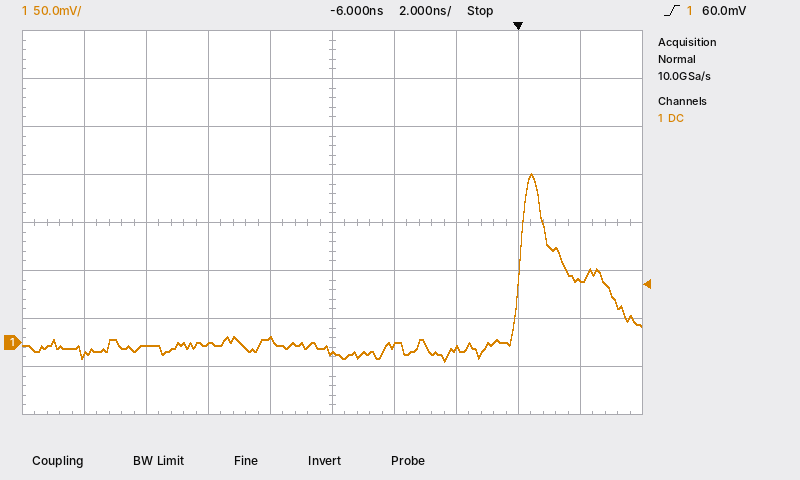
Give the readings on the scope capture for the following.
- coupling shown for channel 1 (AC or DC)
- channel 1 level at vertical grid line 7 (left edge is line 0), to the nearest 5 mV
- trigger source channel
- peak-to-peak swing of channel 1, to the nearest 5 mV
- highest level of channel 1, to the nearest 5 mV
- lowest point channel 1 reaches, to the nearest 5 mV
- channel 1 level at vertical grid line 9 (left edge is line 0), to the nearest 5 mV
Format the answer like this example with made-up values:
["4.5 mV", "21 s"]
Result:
["DC", "-5 mV", "channel 1", "195 mV", "175 mV", "-20 mV", "65 mV"]
